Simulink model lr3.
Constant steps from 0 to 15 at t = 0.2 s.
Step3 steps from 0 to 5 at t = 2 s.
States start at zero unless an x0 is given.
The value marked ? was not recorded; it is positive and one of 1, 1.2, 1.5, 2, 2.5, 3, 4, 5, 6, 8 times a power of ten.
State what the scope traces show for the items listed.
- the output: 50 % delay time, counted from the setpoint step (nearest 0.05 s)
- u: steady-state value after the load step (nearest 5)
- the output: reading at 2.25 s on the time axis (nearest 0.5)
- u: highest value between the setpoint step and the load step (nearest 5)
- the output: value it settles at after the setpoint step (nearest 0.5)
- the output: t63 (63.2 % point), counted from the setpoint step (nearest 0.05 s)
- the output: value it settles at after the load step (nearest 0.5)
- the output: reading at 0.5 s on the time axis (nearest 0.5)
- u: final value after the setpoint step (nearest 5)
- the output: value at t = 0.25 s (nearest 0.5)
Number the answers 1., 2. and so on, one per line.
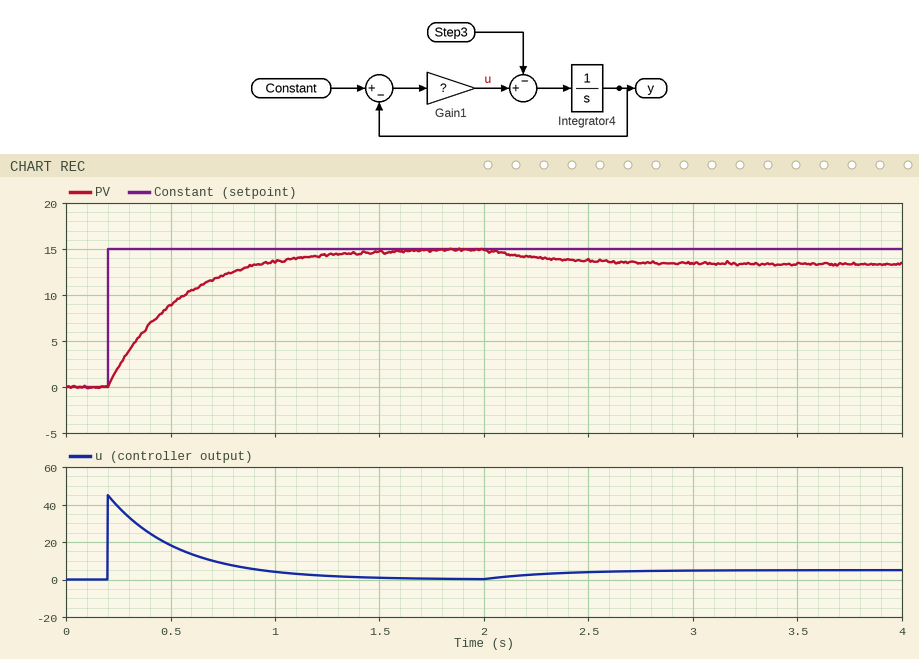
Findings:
1. 0.25 s
2. 5
3. 14.0
4. 45
5. 15.0
6. 0.35 s
7. 13.5
8. 9.0
9. 0
10. 2.0
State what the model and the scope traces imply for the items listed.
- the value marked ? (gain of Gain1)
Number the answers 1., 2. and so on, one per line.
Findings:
1. 3
